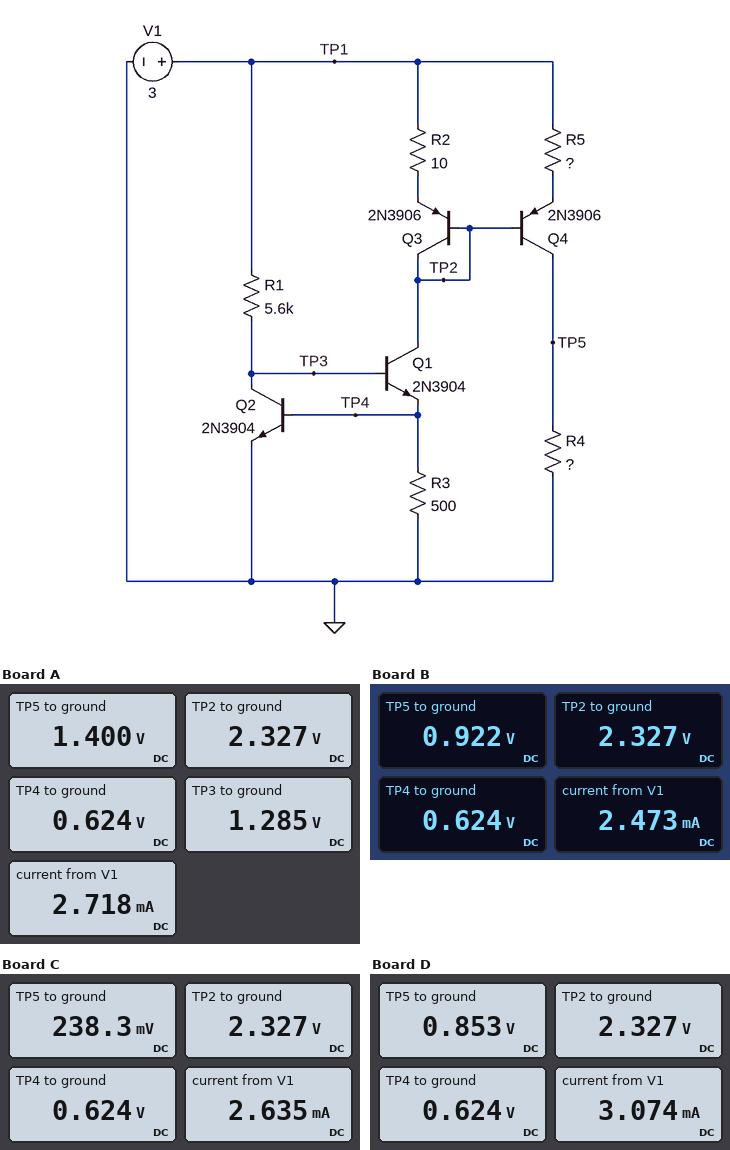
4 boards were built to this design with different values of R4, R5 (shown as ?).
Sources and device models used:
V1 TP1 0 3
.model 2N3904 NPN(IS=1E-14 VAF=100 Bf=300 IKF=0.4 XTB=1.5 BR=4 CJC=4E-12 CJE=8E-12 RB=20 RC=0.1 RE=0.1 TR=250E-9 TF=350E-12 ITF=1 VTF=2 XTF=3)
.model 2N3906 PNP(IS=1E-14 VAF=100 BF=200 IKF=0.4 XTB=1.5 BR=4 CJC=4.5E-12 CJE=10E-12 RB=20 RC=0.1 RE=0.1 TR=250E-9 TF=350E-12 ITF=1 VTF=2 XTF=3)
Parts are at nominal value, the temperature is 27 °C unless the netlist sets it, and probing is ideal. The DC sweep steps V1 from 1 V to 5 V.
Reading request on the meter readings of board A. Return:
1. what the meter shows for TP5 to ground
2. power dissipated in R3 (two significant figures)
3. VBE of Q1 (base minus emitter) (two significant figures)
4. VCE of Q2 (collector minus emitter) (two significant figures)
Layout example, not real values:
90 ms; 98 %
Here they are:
1.400 V; 780 µW; 660 mV; 1.3 V
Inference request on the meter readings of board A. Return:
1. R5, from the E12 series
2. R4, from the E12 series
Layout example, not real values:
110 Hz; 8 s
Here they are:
12 Ω; 1.2 kΩ
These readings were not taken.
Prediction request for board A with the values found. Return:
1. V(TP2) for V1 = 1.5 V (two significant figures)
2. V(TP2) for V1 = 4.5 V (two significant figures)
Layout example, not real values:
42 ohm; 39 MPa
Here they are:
830 mV; 3.8 V
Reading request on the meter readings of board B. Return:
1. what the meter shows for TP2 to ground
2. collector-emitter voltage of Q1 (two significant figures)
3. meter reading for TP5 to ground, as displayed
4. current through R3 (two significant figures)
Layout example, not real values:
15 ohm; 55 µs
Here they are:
2.327 V; 1.7 V; 0.922 V; 1.2 mA
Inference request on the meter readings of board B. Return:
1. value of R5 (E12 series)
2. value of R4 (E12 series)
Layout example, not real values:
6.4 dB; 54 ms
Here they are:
22 Ω; 1 kΩ
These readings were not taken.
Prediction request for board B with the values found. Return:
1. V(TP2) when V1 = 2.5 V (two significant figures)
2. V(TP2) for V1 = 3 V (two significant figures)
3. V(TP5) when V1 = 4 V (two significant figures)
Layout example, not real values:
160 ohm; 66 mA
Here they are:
1.8 V; 2.3 V; 940 mV
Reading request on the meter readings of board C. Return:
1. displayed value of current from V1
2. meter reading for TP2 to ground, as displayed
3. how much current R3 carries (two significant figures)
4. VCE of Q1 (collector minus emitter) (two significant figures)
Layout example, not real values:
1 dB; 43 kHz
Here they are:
2.635 mA; 2.327 V; 1.2 mA; 1.7 V
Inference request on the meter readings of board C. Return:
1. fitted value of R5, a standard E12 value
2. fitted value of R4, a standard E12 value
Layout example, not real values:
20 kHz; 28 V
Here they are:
15 Ω; 220 Ω
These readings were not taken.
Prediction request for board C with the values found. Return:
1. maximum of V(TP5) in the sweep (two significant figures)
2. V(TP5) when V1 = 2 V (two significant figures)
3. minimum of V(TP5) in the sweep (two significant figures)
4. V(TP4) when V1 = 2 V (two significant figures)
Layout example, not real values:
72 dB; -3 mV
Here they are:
250 mV; 230 mV; 110 mV; 600 mV
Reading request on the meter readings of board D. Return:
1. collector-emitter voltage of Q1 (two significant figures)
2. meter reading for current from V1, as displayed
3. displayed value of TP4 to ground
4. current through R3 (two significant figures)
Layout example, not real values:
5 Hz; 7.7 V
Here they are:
1.7 V; 3.074 mA; 0.624 V; 1.2 mA
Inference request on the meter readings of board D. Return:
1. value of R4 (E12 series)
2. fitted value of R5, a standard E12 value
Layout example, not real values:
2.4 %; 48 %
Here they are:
560 Ω; 4.7 Ω
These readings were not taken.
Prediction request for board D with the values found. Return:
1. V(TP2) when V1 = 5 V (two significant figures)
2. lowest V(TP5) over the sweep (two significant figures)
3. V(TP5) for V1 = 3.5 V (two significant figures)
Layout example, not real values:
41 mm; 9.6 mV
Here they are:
4.3 V; 340 mV; 870 mV
